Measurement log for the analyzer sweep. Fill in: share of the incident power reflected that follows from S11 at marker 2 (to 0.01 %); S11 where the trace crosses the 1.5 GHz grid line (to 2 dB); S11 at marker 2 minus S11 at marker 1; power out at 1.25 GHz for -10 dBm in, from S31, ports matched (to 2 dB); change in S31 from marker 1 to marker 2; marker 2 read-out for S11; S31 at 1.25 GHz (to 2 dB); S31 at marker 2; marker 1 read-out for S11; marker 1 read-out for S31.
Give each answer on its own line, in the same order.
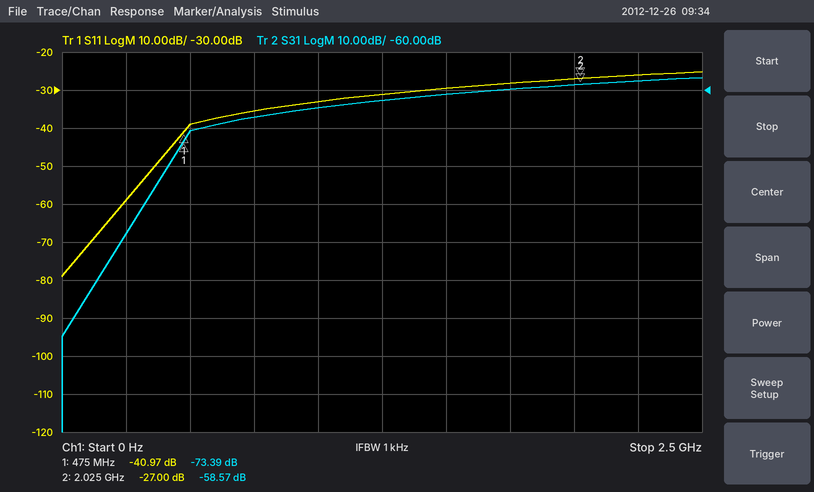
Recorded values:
0.20 %
-30 dB
13.97 dB
-72 dBm
14.82 dB
-27.00 dB
-62 dB
-58.57 dB
-40.97 dB
-73.39 dB
